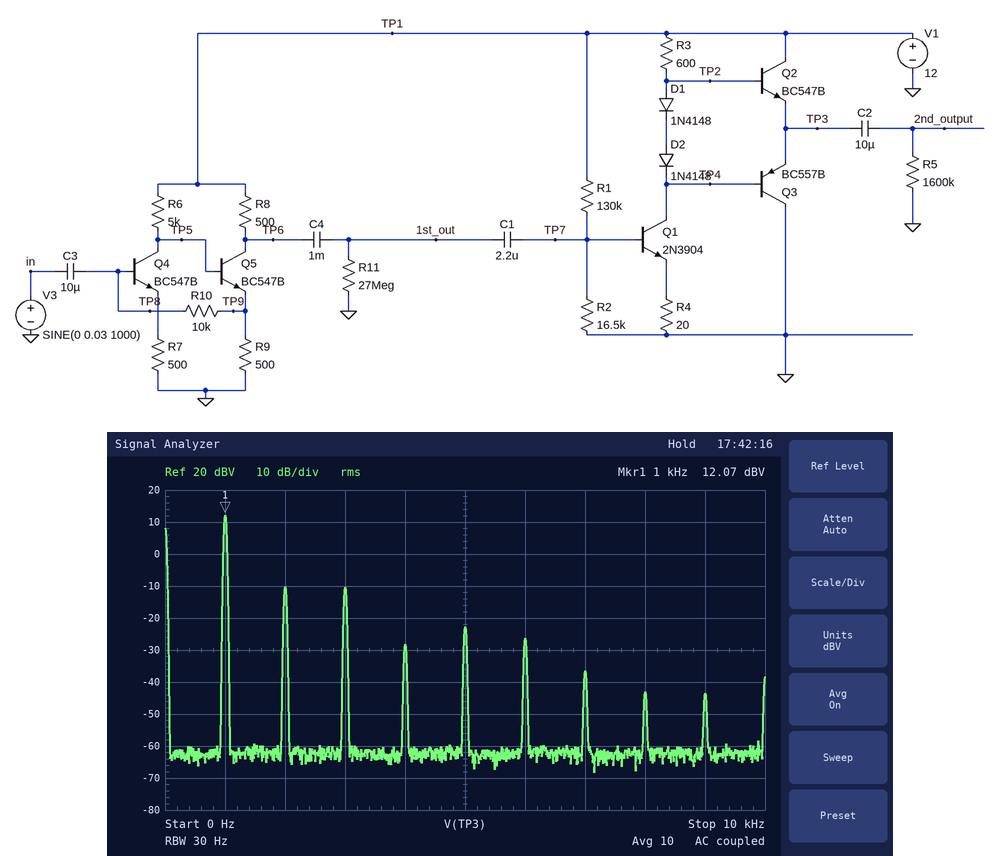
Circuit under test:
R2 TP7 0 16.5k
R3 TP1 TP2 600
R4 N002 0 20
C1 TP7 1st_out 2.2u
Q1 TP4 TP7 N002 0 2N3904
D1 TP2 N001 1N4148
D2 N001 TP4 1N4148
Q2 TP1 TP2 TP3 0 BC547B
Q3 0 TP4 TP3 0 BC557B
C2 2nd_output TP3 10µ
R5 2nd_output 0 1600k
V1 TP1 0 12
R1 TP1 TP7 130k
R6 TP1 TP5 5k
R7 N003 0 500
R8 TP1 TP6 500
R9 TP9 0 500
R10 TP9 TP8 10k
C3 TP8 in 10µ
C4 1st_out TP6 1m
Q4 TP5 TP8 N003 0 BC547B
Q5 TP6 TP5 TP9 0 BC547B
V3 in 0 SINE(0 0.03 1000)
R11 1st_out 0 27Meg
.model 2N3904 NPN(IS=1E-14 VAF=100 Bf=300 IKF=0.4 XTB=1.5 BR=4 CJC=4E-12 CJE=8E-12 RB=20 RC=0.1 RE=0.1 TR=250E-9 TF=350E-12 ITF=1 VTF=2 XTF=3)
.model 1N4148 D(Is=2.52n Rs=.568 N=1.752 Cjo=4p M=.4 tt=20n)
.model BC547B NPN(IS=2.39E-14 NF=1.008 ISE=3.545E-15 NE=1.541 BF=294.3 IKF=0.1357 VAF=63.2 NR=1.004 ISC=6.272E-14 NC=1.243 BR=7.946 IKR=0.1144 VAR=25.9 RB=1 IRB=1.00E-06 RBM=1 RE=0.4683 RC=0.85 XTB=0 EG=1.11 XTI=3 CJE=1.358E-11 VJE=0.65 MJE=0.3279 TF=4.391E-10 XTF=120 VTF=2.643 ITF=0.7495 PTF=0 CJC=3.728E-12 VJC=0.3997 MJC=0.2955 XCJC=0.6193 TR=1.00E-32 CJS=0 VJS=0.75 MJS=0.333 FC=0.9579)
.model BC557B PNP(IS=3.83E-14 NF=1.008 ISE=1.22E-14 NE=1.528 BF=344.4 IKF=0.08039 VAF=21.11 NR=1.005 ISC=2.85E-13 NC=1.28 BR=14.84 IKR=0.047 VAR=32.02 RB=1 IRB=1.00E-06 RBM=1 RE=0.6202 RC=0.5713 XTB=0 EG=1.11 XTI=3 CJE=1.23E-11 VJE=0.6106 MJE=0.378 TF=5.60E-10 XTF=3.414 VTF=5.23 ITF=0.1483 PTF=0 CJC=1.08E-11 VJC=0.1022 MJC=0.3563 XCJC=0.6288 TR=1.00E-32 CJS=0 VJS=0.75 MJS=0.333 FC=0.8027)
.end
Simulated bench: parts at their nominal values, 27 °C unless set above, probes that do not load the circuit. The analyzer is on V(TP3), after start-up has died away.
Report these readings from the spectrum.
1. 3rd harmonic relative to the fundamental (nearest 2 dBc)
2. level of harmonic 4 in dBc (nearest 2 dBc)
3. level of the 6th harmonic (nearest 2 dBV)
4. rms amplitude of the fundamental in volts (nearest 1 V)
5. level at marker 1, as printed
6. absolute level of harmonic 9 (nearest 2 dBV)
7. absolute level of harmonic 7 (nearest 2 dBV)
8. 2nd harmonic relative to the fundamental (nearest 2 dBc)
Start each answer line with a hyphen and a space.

- -22 dBc
- -40 dBc
- -26 dBV
- 4 V
- 12.07 dBV
- -44 dBV
- -36 dBV
- -22 dBc
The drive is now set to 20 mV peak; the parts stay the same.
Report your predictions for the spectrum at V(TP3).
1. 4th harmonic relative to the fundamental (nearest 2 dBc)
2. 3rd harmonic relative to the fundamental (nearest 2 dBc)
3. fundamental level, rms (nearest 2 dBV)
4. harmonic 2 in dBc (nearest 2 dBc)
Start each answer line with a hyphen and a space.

- -56 dBc
- -42 dBc
- 10 dBV
- -32 dBc
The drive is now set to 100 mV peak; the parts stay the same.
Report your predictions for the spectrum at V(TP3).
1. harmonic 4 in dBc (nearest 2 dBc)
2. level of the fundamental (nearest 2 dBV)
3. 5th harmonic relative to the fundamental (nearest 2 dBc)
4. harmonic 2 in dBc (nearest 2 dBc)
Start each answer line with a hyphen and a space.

- -16 dBc
- 12 dBV
- -16 dBc
- -6 dBc
